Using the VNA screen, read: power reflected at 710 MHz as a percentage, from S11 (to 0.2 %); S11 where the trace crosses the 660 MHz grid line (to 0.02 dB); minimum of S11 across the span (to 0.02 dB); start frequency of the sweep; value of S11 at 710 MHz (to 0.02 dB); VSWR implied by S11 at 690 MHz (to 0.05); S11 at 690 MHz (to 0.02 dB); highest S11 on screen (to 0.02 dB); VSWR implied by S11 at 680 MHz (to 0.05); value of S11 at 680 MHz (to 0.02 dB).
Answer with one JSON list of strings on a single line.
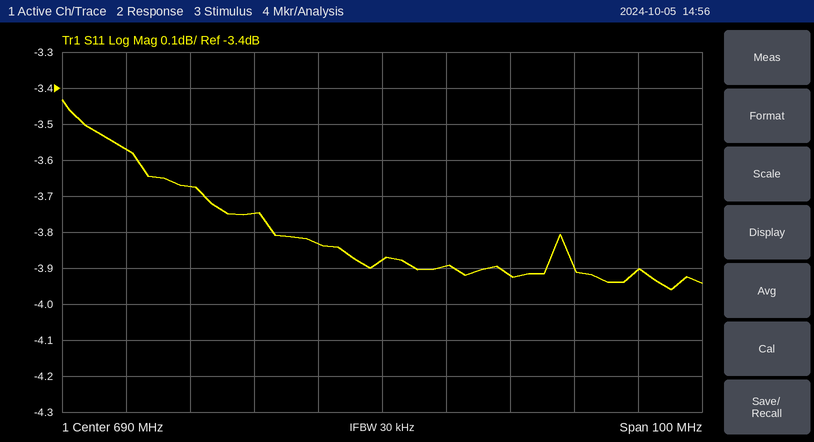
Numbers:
["40.6 %", "-3.68 dB", "-3.96 dB", "640 MHz", "-3.92 dB", "4.55", "-3.88 dB", "-3.44 dB", "4.60", "-3.84 dB"]
